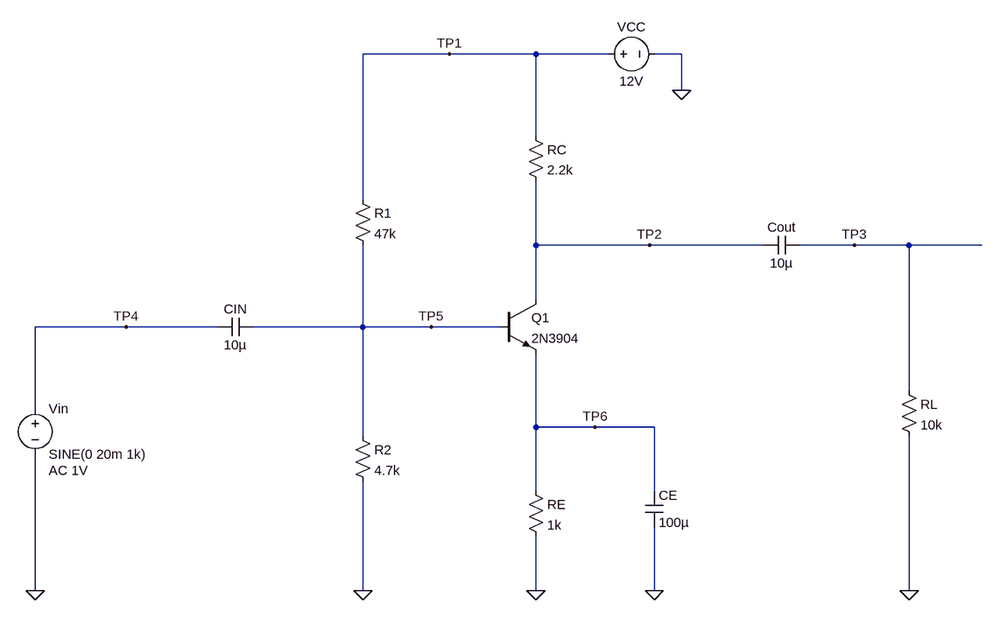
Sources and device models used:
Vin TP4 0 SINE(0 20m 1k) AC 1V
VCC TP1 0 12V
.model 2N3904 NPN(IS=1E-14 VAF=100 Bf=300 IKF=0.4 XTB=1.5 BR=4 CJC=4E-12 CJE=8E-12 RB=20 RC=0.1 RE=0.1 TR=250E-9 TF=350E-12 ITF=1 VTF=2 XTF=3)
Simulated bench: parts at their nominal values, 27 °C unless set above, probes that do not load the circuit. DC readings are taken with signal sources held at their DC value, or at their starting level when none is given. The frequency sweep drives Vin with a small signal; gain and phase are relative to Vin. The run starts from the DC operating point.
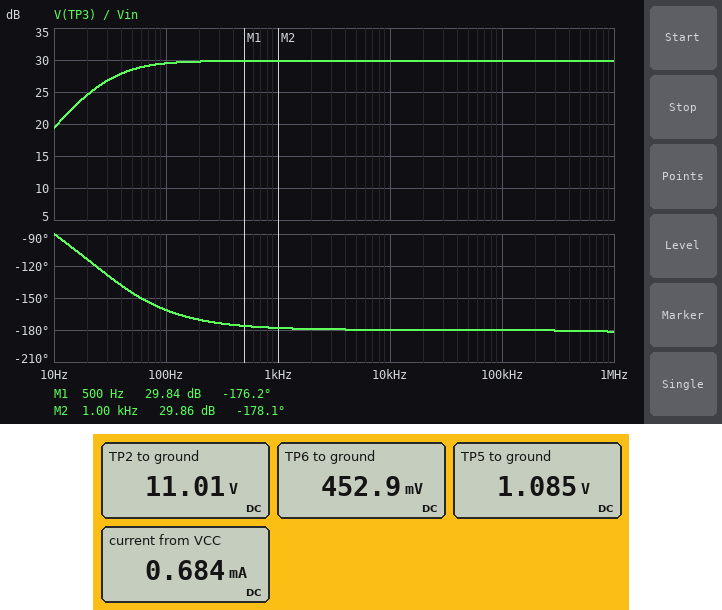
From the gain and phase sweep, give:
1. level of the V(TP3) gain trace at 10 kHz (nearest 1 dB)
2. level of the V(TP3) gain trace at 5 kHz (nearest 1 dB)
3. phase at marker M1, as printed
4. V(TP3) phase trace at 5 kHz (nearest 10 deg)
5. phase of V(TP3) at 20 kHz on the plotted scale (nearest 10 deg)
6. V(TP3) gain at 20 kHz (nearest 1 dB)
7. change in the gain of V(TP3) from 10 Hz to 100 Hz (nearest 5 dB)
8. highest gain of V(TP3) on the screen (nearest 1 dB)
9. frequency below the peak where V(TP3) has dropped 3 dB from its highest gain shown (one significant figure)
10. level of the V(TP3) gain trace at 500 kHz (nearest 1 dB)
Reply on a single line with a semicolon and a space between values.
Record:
30 dB; 30 dB; -176.2 deg; -180 deg; -180 deg; 30 dB; 10 dB; 30 dB; 30 Hz; 30 dB
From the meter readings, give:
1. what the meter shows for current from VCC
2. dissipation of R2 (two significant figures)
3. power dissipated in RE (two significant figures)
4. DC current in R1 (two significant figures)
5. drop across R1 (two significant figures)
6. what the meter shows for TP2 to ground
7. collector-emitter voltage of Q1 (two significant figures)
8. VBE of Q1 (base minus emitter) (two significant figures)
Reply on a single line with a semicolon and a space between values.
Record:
0.684 mA; 250 µW; 210 µW; 230 µA; 11 V; 11.01 V; 11 V; 630 mV
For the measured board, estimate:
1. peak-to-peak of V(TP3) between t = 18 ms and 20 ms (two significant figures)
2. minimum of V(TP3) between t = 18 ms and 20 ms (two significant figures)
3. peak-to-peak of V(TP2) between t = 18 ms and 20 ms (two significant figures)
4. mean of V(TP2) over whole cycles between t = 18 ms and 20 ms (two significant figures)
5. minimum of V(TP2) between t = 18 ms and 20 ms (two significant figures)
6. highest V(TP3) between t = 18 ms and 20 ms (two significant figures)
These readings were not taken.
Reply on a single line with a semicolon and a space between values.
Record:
1.2 V; -710 mV; 1.2 V; 11 V; 10 V; 490 mV
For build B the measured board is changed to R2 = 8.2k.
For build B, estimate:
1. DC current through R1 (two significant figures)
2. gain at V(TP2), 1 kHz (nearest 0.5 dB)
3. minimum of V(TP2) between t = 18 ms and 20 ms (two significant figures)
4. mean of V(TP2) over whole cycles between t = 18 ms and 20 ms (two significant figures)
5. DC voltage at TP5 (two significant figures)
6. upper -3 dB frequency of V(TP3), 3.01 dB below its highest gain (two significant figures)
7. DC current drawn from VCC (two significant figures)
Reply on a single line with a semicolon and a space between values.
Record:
220 µA; 37.5 dB; 7.9 V; 9.6 V; 1.8 V; 26 MHz; 1.3 mA
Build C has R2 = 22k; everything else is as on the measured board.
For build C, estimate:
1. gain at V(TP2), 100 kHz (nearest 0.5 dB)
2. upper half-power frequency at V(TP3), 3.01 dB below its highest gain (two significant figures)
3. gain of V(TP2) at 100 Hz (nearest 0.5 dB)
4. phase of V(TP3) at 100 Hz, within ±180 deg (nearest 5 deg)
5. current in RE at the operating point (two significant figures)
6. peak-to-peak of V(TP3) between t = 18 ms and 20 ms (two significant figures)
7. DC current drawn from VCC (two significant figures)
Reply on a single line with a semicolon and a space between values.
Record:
45.5 dB; 10 MHz; 39.5 dB; -120 deg; 3.0 mA; 5.5 V; 3.2 mA
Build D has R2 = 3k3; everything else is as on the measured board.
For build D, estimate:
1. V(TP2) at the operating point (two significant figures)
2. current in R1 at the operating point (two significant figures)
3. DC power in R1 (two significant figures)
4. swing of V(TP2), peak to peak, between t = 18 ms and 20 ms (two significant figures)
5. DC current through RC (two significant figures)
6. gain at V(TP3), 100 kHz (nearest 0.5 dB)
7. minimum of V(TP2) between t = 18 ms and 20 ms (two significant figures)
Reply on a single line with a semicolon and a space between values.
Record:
12 V; 240 µA; 2.7 mW; 490 mV; 180 µA; 22.0 dB; 11 V
